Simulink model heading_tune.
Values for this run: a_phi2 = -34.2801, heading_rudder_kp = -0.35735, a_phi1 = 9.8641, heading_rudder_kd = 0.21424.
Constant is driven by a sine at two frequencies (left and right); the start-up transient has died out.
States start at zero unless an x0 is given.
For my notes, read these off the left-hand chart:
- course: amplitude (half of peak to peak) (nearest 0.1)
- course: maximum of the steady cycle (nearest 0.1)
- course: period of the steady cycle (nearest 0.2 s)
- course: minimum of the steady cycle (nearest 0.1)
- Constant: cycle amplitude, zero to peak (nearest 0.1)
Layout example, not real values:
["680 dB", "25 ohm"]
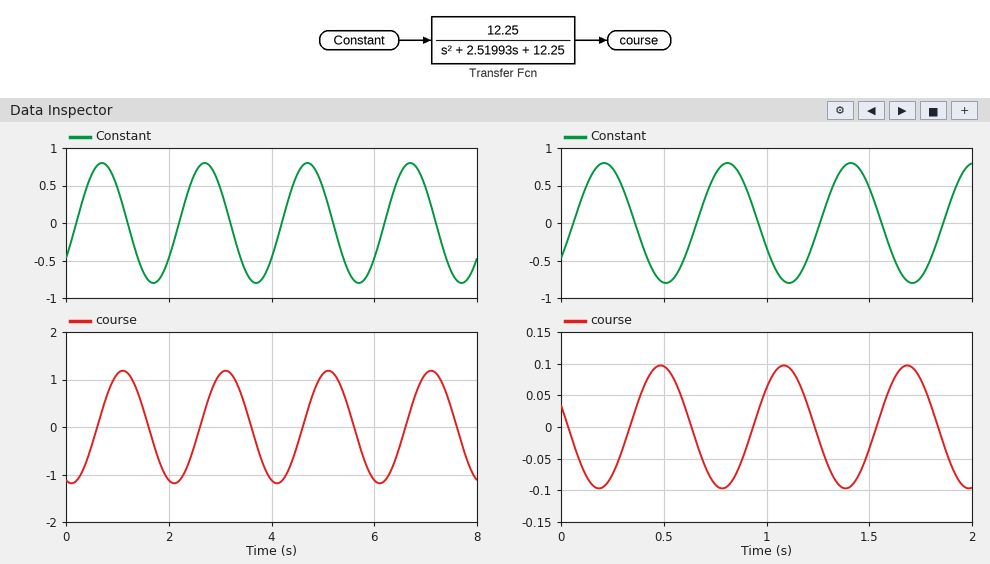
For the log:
["1.2", "1.2", "2.0 s", "-1.2", "0.8"]
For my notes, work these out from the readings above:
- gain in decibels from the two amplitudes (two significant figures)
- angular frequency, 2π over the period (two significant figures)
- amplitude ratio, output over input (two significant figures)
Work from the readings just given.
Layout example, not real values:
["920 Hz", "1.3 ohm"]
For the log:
["3.5 dB", "3.1 rad/s", "1.5"]
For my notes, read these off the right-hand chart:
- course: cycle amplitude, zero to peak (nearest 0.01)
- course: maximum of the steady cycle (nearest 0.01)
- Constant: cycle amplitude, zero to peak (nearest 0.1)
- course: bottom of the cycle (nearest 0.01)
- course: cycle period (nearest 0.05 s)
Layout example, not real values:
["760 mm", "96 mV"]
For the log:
["0.10", "0.10", "0.8", "-0.10", "0.60 s"]
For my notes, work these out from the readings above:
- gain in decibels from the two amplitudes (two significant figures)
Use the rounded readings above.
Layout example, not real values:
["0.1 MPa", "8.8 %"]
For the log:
["-18 dB"]
